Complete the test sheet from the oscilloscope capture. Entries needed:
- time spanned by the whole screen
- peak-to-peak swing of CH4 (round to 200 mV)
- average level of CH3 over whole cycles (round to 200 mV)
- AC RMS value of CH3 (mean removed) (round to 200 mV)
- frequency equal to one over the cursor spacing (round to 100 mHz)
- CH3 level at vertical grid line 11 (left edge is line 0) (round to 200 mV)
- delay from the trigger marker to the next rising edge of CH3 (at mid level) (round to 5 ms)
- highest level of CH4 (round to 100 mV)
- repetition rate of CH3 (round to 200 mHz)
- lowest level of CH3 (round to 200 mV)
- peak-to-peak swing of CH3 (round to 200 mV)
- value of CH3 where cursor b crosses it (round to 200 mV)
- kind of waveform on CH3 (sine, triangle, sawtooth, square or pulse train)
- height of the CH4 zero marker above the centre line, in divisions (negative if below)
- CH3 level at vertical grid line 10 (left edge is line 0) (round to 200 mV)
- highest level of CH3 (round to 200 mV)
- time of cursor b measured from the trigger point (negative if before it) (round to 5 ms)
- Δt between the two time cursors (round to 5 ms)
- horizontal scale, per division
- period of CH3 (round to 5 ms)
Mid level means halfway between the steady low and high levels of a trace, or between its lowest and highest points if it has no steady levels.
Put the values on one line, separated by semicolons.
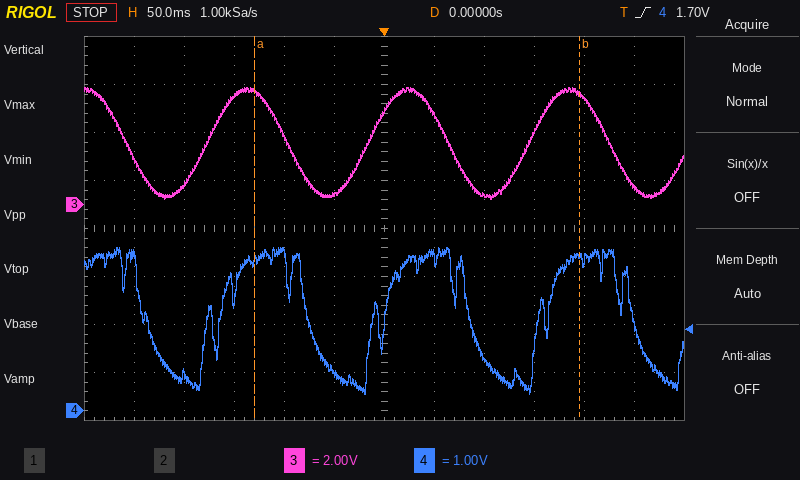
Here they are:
600 ms; 3.0 V; 2.6 V; 1.6 V; 3.1 Hz; 800 mV; 145 ms; 3.4 V; 6.2 Hz; 200 mV; 4.6 V; 4.6 V; sine; -3.8 div; 4.4 V; 4.8 V; +195 ms; 325 ms; 50 ms; 160 ms
